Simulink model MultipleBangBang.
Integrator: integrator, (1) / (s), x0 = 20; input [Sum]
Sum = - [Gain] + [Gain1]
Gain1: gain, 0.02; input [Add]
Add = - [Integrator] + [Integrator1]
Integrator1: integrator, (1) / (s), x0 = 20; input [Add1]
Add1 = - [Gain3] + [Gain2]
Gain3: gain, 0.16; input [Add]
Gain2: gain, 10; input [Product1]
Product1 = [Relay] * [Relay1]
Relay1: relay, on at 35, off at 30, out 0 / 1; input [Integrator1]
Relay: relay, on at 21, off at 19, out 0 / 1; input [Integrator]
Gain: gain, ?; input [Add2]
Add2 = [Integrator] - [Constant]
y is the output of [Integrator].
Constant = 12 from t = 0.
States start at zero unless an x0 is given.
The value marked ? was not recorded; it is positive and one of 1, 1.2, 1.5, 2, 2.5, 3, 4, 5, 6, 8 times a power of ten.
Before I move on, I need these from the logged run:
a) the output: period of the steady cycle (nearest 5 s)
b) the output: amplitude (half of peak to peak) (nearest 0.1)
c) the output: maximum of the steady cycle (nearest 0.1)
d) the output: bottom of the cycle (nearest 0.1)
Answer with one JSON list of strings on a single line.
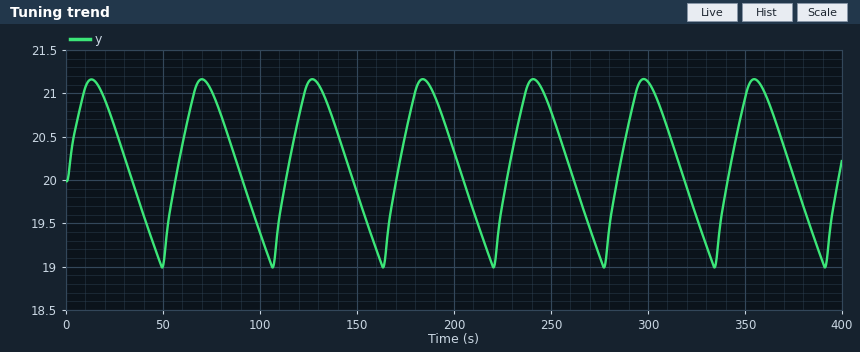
["55 s", "1.1", "21.2", "19.0"]
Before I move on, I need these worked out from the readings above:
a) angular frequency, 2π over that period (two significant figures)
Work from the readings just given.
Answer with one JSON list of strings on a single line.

["0.11 rad/s"]
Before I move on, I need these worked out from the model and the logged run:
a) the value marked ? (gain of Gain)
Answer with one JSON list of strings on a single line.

["0.01"]
